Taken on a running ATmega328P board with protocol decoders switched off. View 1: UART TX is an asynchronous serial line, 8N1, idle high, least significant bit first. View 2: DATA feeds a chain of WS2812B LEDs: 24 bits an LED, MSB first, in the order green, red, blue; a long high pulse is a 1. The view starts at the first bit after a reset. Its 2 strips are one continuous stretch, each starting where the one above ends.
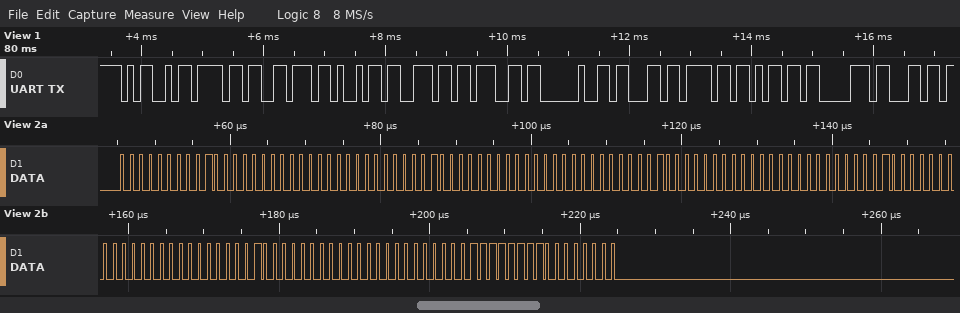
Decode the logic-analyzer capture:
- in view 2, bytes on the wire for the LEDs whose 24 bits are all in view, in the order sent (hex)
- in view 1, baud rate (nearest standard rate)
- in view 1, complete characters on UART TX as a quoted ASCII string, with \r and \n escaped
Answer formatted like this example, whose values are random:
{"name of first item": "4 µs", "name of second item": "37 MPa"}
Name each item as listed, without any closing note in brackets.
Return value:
{"in view 2, bytes on the wire for the LEDs whose 24 bits are all in view, in the order sent": "00 40 00 00 40 00 00 40 00 00 40 00 00 40 00 00 FF 00", "in view 1, baud rate": "9600 baud", "in view 1, complete characters on UART TX as a quoted ASCII string, with \\r and \\n escaped": "\"Moving compl\""}
